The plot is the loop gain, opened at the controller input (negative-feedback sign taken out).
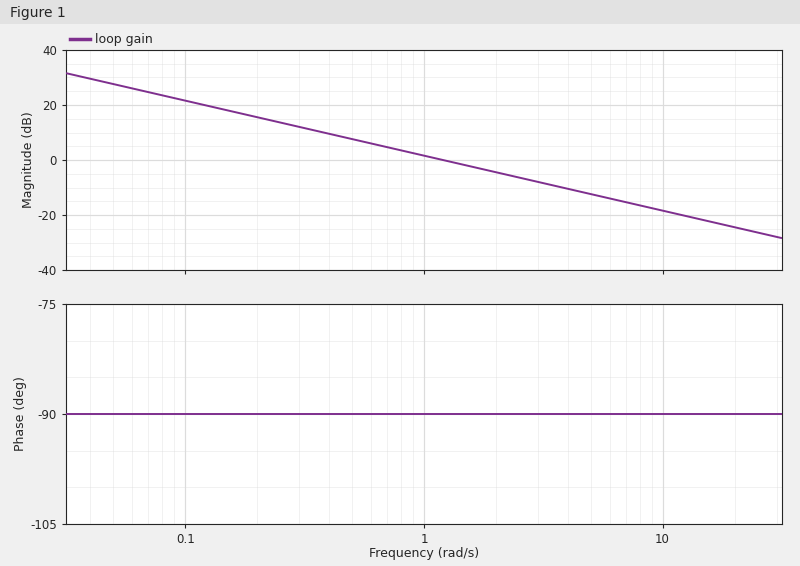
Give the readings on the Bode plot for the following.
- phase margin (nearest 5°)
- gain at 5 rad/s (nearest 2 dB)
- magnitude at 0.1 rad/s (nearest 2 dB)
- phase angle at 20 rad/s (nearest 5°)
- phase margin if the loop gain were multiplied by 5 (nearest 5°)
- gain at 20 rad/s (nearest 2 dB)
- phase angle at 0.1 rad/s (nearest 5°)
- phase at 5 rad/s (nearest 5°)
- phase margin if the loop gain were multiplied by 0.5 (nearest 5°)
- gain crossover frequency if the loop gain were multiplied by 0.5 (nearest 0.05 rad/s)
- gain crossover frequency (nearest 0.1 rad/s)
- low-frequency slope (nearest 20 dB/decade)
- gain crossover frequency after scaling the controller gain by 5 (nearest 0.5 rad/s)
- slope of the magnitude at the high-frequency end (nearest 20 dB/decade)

90°
-12 dB
22 dB
-90°
90°
-24 dB
-90°
-90°
90°
0.60 rad/s
1.2 rad/s
-20 dB/decade
6.0 rad/s
-20 dB/decade
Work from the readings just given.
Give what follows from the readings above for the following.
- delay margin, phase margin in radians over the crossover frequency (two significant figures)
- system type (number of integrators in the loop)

1.3 s
1
